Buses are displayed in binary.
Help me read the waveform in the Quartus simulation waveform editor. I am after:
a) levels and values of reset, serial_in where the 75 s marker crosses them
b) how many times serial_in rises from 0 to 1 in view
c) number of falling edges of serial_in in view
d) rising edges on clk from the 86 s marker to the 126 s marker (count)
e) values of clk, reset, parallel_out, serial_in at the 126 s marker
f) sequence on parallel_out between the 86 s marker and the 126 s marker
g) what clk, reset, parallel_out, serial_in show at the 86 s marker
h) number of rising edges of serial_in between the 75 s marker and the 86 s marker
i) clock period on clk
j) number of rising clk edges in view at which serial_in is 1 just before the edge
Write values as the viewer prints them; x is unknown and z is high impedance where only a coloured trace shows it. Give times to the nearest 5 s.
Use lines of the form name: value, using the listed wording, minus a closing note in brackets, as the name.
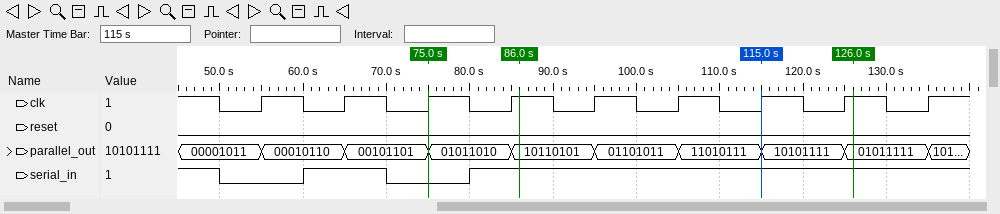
levels and values of reset, serial_in where the 75 s marker crosses them: reset=0, serial_in=0
how many times serial_in rises from 0 to 1 in view: 2
number of falling edges of serial_in in view: 2
rising edges on clk from the 86 s marker to the 126 s marker: 4
values of clk, reset, parallel_out, serial_in at the 126 s marker: clk=1, reset=0, parallel_out=01011111, serial_in=1
sequence on parallel_out between the 86 s marker and the 126 s marker: 10110101, 01101011, 11010111, 10101111, 01011111
what clk, reset, parallel_out, serial_in show at the 86 s marker: clk=1, reset=0, parallel_out=10110101, serial_in=1
number of rising edges of serial_in between the 75 s marker and the 86 s marker: 1
clock period on clk: 10 s
number of rising clk edges in view at which serial_in is 1 just before the edge: 7
